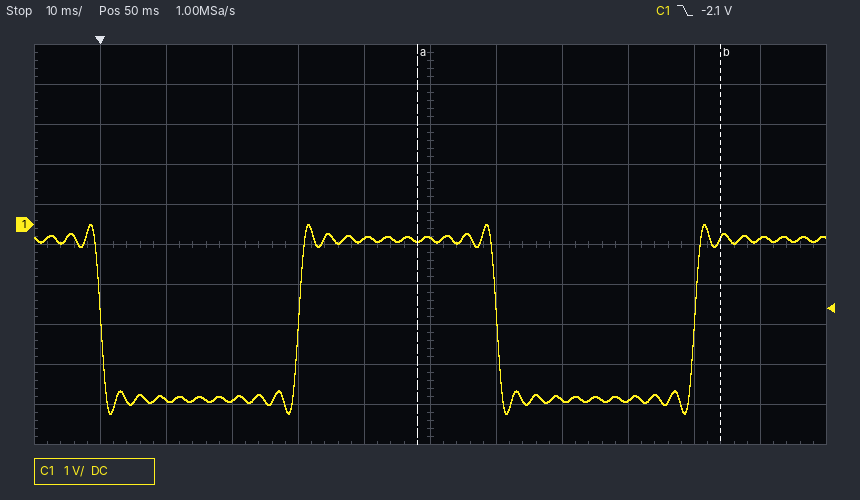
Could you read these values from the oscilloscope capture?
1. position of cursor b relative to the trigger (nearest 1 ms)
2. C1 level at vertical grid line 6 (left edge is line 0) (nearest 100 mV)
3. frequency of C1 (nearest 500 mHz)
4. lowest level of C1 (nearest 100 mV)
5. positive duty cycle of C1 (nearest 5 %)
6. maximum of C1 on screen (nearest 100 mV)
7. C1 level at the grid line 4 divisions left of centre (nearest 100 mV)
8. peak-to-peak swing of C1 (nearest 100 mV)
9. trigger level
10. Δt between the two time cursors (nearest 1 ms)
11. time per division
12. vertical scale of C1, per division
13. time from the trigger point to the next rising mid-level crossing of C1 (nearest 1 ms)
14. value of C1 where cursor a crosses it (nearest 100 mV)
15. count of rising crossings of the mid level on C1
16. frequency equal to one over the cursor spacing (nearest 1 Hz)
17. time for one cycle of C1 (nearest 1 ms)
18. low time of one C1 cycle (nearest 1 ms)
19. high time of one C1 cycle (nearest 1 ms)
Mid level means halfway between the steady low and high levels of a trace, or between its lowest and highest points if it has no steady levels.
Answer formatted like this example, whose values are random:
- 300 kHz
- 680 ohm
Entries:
- +94 ms
- -300 mV
- 16.5 Hz
- -4.7 V
- 50 %
- 0.0 V
- -4.4 V
- 4.7 V
- -2.1 V
- 46 ms
- 10 ms
- 1 V
- 30 ms
- -400 mV
- 2
- 22 Hz
- 60 ms
- 30 ms
- 30 ms
